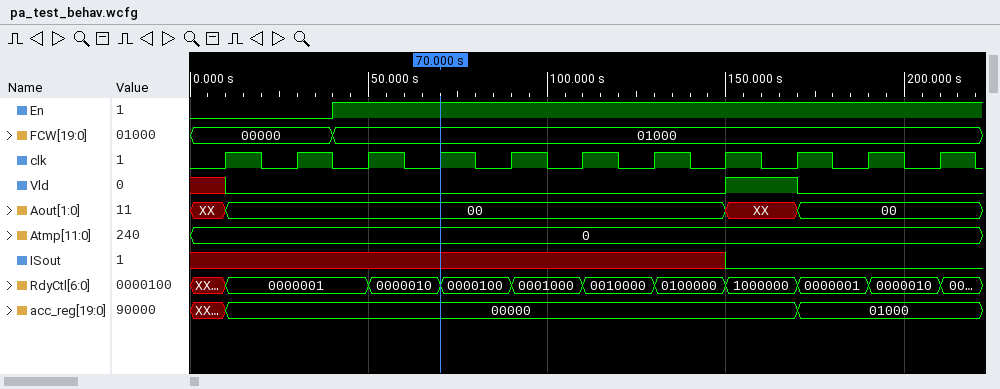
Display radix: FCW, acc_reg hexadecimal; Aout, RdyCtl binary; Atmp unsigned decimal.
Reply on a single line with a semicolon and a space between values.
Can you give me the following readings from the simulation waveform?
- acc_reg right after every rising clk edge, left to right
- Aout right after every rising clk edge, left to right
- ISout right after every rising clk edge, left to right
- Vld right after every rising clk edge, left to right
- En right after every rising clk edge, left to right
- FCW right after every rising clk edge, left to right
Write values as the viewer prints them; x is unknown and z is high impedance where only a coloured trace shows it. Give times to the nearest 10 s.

00000, 00000, 00000, 00000, 00000, 00000, 00000, 00000, 01000, 01000, 01000; 00, 00, 00, 00, 00, 00, 00, XX, 00, 00, 00; x x x x x x x 0 0 0 0; 0 0 0 0 0 0 0 1 0 0 0; 0 0 1 1 1 1 1 1 1 1 1; 00000, 00000, 01000, 01000, 01000, 01000, 01000, 01000, 01000, 01000, 01000
